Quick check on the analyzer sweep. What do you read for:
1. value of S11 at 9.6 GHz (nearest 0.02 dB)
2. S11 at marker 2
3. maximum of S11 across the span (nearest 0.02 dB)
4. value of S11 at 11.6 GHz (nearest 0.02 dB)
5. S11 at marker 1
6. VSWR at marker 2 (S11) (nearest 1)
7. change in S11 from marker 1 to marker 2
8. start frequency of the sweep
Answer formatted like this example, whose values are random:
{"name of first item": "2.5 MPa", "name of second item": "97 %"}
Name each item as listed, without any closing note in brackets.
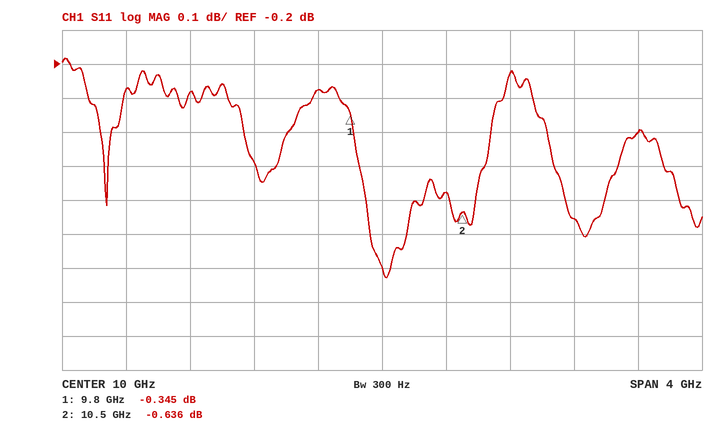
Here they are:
{"value of S11 at 9.6 GHz": "-0.28 dB", "S11 at marker 2": "-0.636 dB", "maximum of S11 across the span": "-0.18 dB", "value of S11 at 11.6 GHz": "-0.40 dB", "S11 at marker 1": "-0.345 dB", "VSWR at marker 2 (S11)": "27", "change in S11 from marker 1 to marker 2": "-0.291 dB", "start frequency of the sweep": "8 GHz"}
